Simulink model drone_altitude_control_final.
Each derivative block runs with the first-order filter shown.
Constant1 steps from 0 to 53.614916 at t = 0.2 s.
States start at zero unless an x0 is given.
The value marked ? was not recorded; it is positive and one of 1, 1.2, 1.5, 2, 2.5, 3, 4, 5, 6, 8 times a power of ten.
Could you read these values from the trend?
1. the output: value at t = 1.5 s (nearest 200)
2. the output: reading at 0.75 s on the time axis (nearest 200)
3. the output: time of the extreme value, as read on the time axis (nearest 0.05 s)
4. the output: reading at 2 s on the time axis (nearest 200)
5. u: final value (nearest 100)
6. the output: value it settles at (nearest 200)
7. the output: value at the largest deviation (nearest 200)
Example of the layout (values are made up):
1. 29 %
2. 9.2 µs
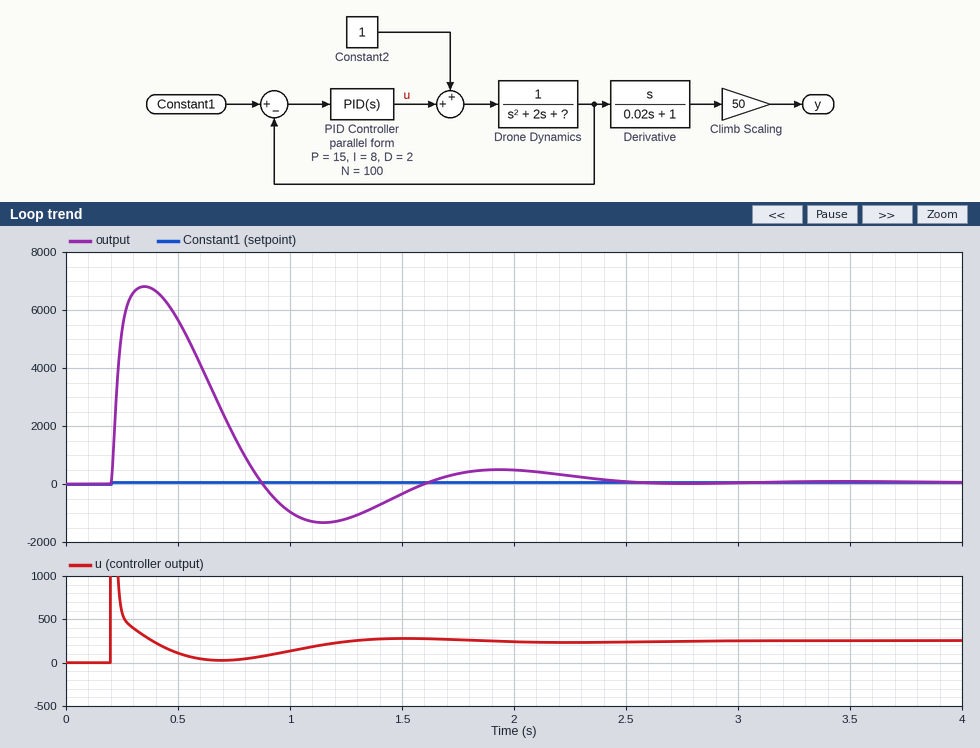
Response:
1. -400
2. 1600
3. 0.35 s
4. 400
5. 300
6. 0
7. 6800
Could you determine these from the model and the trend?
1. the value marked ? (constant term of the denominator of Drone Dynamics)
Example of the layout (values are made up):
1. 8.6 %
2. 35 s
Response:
1. 5
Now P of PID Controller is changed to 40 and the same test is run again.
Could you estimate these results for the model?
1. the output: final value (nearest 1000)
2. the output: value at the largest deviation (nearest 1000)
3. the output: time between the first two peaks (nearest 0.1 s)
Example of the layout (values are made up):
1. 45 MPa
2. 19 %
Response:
1. 0
2. 12000
3. 1.0 s
